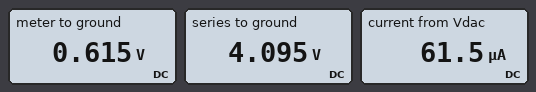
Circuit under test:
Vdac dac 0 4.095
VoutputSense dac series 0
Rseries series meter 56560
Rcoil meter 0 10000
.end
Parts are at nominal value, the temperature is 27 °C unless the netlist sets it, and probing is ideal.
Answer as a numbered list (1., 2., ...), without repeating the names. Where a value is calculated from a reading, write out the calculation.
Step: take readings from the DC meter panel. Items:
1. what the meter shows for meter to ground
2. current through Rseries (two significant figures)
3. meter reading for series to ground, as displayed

1. 0.615 V
2. (4.095 V - 615 mV) / 56.56 kΩ = 62 µA
3. 4.095 V
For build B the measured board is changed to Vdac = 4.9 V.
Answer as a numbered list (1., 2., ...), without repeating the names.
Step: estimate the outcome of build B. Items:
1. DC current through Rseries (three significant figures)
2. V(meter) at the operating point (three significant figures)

1. 73.6 µA
2. 736 mV
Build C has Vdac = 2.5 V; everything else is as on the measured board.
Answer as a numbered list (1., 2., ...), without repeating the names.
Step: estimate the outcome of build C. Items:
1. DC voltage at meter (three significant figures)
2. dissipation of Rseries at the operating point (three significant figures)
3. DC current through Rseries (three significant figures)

1. 376 mV
2. 79.8 µW
3. 37.6 µA
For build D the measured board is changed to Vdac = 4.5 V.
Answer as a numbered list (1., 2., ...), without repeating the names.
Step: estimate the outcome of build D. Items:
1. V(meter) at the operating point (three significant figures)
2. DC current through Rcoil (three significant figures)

1. 676 mV
2. 67.6 µA
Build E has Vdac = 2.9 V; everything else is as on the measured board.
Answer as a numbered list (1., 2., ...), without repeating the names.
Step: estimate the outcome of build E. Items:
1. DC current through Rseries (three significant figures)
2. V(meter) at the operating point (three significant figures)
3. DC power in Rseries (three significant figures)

1. 43.6 µA
2. 436 mV
3. 107 µW
